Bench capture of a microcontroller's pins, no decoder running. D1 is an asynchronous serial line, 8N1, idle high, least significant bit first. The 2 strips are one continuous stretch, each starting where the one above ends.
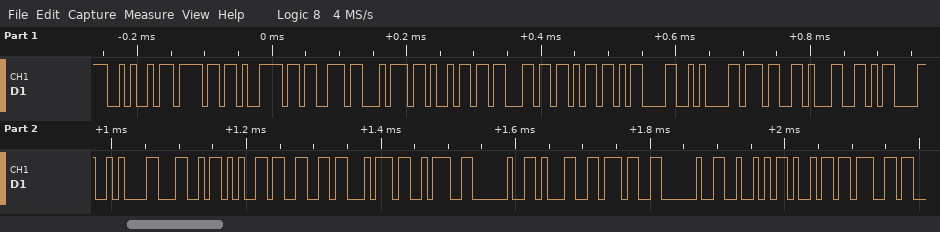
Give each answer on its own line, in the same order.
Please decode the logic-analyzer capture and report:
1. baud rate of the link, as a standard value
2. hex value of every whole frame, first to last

115200 baud
4A 6F 79 73 74 69 63 6B 0D 0A 37 31 0D 0A 4C 65 66 74 3A 20 31 37 20 52 69 67
